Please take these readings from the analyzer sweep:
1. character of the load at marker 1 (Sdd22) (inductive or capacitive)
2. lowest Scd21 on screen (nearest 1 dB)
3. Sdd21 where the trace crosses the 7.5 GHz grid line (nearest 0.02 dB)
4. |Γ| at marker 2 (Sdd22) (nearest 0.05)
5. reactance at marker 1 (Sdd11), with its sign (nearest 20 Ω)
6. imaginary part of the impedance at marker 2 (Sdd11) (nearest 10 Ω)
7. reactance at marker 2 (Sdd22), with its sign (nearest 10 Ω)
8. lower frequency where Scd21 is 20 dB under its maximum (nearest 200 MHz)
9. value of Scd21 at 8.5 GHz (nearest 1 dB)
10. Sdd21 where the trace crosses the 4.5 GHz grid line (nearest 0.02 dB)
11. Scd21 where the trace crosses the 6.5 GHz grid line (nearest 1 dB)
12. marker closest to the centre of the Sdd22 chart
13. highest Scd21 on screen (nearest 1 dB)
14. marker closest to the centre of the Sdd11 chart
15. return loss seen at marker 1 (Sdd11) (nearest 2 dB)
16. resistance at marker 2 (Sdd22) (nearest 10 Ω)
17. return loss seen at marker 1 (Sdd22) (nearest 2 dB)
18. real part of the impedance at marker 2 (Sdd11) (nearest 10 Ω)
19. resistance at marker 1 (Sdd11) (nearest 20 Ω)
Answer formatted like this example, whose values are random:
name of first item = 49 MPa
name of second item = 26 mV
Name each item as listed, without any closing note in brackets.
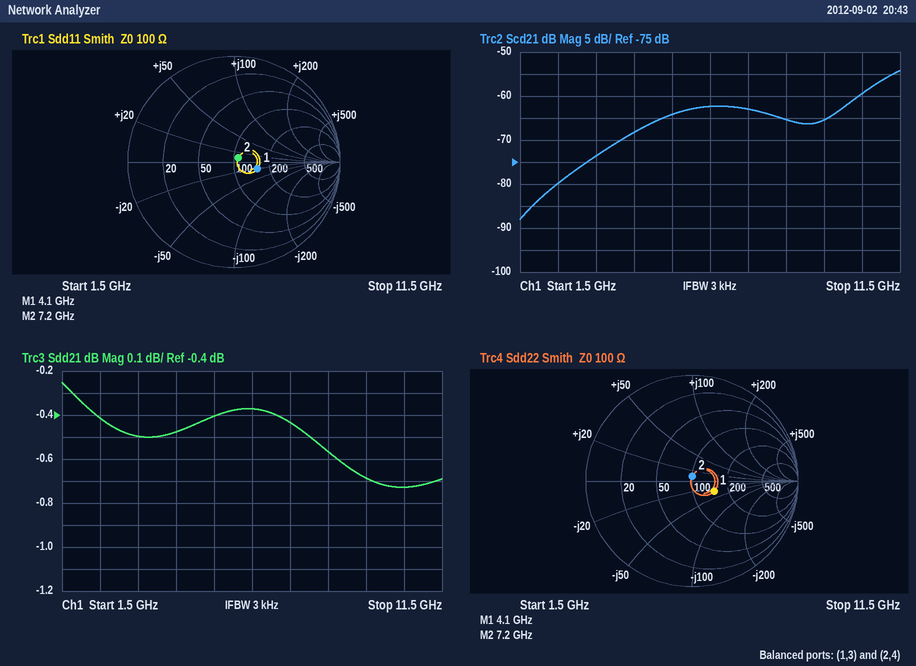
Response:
character of the load at marker 1 (Sdd22) = capacitive
lowest Scd21 on screen = -88 dB
Sdd21 where the trace crosses the 7.5 GHz grid line = -0.44 dB
|Γ| at marker 2 (Sdd22) = 0.05
reactance at marker 1 (Sdd11), with its sign = -20 Ω
imaginary part of the impedance at marker 2 (Sdd11) = +10 Ω
reactance at marker 2 (Sdd22), with its sign = +10 Ω
lower frequency where Scd21 is 20 dB under its maximum = 3.4 GHz
value of Scd21 at 8.5 GHz = -65 dB
Sdd21 where the trace crosses the 4.5 GHz grid line = -0.48 dB
Scd21 where the trace crosses the 6.5 GHz grid line = -62 dB
marker closest to the centre of the Sdd22 chart = marker 2
highest Scd21 on screen = -54 dB
marker closest to the centre of the Sdd11 chart = marker 2
return loss seen at marker 1 (Sdd11) = 12 dB
resistance at marker 2 (Sdd22) = 100 Ω
return loss seen at marker 1 (Sdd22) = 12 dB
real part of the impedance at marker 2 (Sdd11) = 110 Ω
resistance at marker 1 (Sdd11) = 160 Ω
